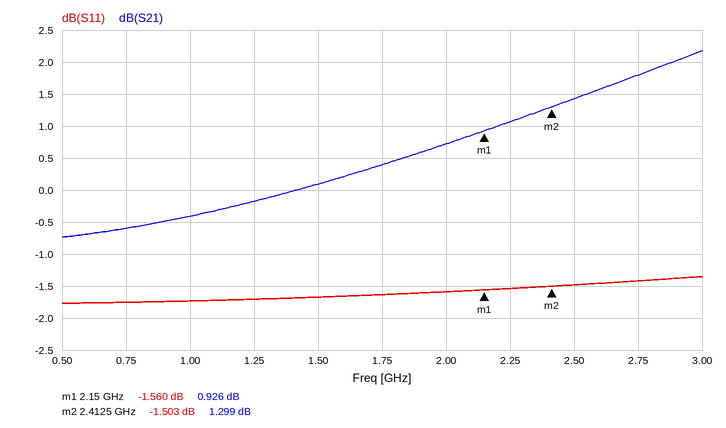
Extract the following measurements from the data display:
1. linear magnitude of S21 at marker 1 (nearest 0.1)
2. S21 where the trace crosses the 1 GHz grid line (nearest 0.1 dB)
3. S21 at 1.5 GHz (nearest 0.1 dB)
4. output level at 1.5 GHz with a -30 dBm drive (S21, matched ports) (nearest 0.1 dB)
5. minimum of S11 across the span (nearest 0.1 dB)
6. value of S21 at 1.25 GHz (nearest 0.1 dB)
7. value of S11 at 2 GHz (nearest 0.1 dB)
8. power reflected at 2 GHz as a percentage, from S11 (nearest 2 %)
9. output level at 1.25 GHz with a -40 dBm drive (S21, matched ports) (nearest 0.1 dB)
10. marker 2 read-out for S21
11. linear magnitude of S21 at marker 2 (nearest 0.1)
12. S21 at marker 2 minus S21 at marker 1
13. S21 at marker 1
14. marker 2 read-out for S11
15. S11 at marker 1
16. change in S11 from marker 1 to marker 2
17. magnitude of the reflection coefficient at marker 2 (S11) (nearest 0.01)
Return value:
1.1
-0.4 dB
0.1 dB
-29.9 dBm
-1.8 dB
-0.2 dB
-1.6 dB
70 %
-40.2 dBm
1.299 dB
1.2
0.373 dB
0.926 dB
-1.503 dB
-1.560 dB
0.057 dB
0.84
